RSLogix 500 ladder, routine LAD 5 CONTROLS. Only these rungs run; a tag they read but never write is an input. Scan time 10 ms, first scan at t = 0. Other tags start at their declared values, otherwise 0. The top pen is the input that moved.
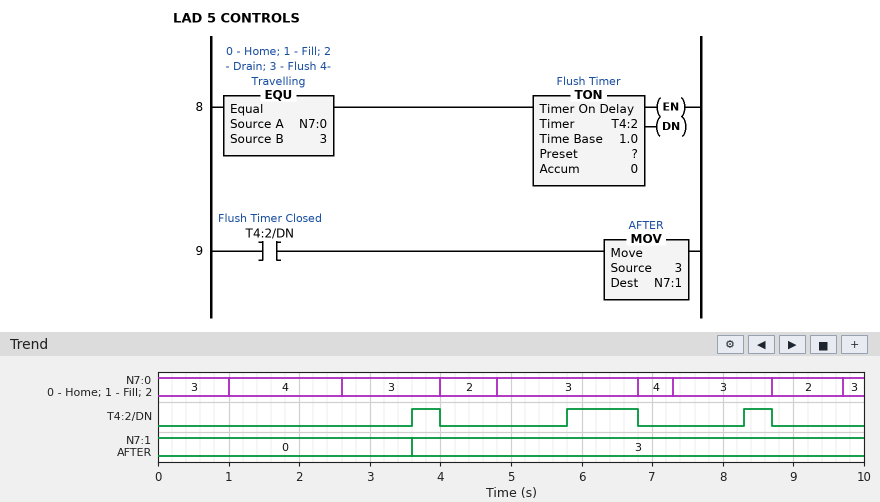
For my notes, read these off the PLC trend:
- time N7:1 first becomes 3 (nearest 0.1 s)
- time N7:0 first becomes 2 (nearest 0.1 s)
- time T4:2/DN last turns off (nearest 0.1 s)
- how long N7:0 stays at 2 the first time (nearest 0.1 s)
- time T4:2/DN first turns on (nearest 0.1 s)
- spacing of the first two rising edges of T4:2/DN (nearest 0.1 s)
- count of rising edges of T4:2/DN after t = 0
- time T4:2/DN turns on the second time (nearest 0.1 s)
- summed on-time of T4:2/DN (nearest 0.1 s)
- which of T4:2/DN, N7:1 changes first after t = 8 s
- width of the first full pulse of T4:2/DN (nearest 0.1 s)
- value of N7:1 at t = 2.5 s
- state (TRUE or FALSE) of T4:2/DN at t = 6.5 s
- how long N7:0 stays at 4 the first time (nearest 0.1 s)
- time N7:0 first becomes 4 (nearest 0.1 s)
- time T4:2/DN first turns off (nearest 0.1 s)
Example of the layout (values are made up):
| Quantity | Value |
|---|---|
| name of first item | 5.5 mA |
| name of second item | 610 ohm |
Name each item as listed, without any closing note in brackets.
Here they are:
| Quantity | Value |
|---|---|
| time N7:1 first becomes 3 | 3.6 s |
| time N7:0 first becomes 2 | 4.0 s |
| time T4:2/DN last turns off | 8.7 s |
| how long N7:0 stays at 2 the first time | 0.8 s |
| time T4:2/DN first turns on | 3.6 s |
| spacing of the first two rising edges of T4:2/DN | 2.2 s |
| count of rising edges of T4:2/DN after t = 0 | 3 |
| time T4:2/DN turns on the second time | 5.8 s |
| summed on-time of T4:2/DN | 1.8 s |
| which of T4:2/DN, N7:1 changes first after t = 8 s | T4:2/DN |
| width of the first full pulse of T4:2/DN | 0.4 s |
| value of N7:1 at t = 2.5 s | 0 |
| state (TRUE or FALSE) of T4:2/DN at t = 6.5 s | TRUE |
| how long N7:0 stays at 4 the first time | 1.6 s |
| time N7:0 first becomes 4 | 1.0 s |
| time T4:2/DN first turns off | 4.0 s |
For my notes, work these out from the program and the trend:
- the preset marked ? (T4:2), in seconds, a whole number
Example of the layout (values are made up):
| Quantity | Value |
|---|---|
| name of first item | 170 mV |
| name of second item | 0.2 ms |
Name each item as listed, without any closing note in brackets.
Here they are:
| Quantity | Value |
|---|---|
| the preset marked ? (T4:2), in seconds, a whole number | 1 s |
